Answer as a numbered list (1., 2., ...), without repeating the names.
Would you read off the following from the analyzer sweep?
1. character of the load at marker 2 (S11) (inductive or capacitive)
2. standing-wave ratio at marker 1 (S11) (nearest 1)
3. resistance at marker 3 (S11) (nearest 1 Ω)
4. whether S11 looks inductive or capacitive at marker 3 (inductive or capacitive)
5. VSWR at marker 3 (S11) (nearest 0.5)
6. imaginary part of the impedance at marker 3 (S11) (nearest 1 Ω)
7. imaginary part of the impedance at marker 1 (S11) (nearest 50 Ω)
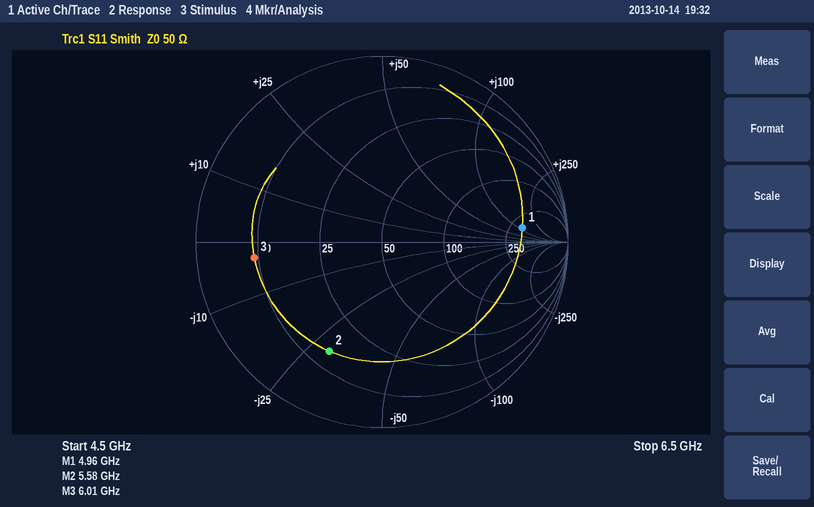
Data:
1. capacitive
2. 7
3. 9 Ω
4. capacitive
5. 5.5
6. -3 Ω
7. +100 Ω
